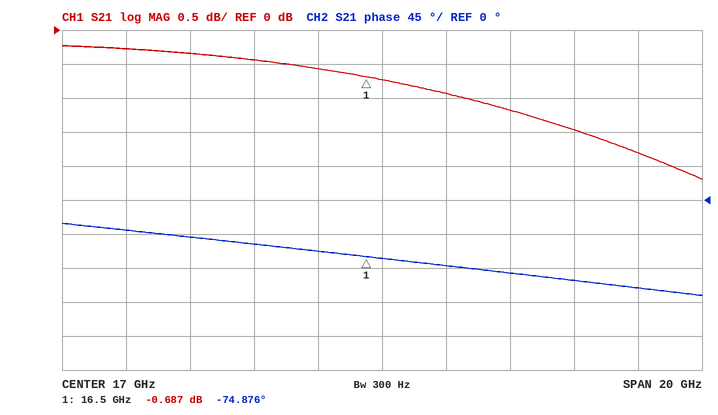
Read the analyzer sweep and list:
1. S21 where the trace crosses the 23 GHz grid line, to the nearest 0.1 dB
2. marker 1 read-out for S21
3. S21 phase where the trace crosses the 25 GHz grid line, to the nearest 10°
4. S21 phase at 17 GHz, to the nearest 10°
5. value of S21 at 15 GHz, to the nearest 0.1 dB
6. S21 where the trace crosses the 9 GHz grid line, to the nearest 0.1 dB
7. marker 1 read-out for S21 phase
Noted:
-1.5 dB
-0.687 dB
-120°
-80°
-0.6 dB
-0.3 dB
-74.876°
